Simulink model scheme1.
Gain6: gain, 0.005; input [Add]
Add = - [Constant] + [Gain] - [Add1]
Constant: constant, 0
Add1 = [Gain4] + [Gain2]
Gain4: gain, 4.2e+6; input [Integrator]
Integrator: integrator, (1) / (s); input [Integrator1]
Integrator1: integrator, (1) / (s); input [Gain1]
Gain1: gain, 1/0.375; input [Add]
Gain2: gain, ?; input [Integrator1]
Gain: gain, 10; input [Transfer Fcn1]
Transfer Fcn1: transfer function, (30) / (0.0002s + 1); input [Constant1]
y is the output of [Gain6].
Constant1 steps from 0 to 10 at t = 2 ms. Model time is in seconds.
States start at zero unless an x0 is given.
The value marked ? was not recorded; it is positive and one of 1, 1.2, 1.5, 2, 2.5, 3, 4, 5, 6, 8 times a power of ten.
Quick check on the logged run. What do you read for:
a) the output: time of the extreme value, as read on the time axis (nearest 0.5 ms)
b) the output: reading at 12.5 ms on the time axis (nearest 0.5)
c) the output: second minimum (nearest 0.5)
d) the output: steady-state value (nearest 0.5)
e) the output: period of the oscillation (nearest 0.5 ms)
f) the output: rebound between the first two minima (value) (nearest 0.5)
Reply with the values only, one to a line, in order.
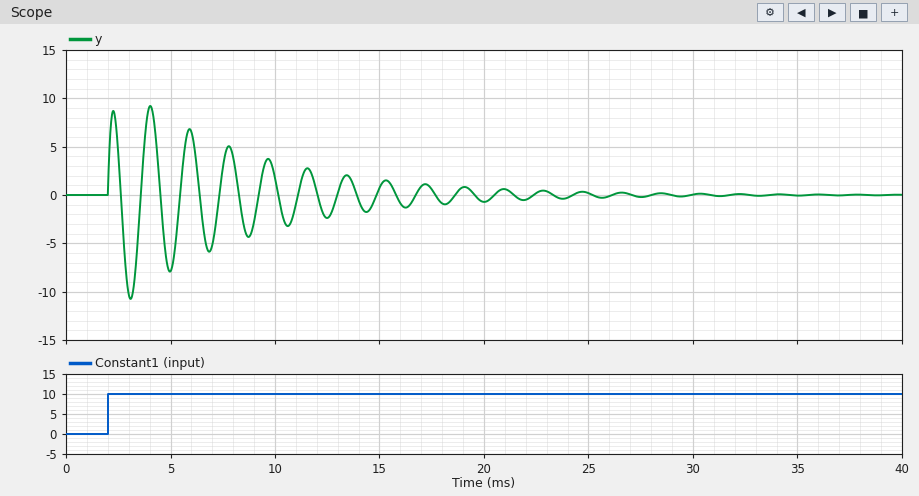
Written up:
3.0 ms
-2.5
-8.0
0.0
2.0 ms
9.0
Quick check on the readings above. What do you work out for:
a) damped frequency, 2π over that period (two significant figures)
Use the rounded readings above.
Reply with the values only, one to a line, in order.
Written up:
3.1 rad/ms
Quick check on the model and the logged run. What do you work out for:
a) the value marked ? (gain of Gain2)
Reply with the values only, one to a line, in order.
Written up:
120
